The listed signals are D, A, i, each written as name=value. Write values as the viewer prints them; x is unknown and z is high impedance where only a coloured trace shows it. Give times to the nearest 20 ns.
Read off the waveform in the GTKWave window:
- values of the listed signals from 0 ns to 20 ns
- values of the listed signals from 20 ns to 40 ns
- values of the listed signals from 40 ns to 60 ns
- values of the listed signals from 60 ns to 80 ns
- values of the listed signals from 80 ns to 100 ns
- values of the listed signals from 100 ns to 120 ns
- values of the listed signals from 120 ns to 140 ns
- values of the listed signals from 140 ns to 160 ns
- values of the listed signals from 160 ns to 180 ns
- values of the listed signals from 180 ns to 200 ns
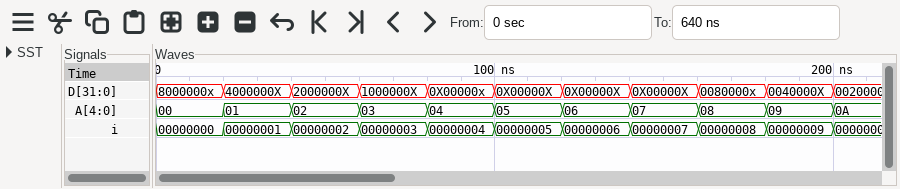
D=8000000x, A=00, i=00000000
D=4000000X, A=01, i=00000001
D=2000000X, A=02, i=00000002
D=1000000X, A=03, i=00000003
D=0X00000x, A=04, i=00000004
D=0X00000X, A=05, i=00000005
D=0X00000X, A=06, i=00000006
D=0X00000X, A=07, i=00000007
D=0080000x, A=08, i=00000008
D=0040000X, A=09, i=00000009
